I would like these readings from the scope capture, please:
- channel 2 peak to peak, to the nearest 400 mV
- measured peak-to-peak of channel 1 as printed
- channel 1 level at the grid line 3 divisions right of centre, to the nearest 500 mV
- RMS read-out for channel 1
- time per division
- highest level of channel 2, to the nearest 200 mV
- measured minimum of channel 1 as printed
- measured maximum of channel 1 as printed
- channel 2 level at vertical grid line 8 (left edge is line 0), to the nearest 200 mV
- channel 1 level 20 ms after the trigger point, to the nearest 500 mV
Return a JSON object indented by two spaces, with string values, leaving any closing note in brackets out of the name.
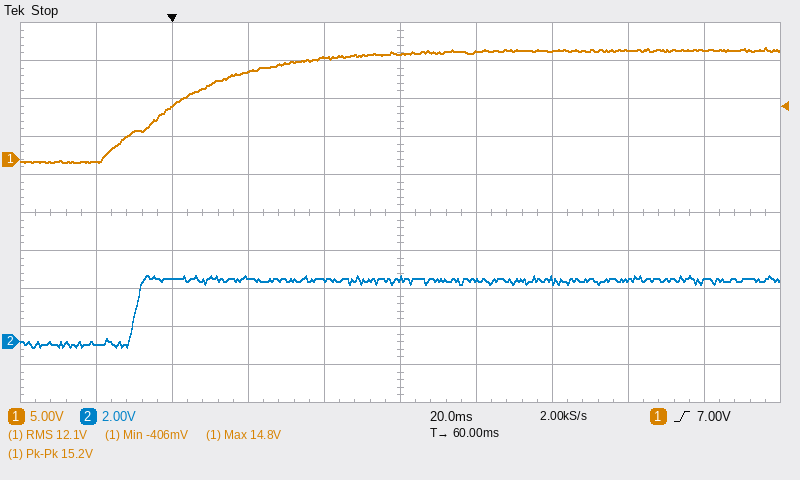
{
  "channel 2 peak to peak, to the nearest 400 mV": "3.6 V",
  "measured peak-to-peak of channel 1 as printed": "15.2 V",
  "channel 1 level at the grid line 3 divisions right of centre, to the nearest 500 mV": "14.5 V",
  "RMS read-out for channel 1": "12.1 V",
  "time per division": "20 ms",
  "highest level of channel 2, to the nearest 200 mV": "3.4 V",
  "measured minimum of channel 1 as printed": "-406 mV",
  "measured maximum of channel 1 as printed": "14.8 V",
  "channel 2 level at vertical grid line 8 (left edge is line 0), to the nearest 200 mV": "3.2 V",
  "channel 1 level 20 ms after the trigger point, to the nearest 500 mV": "11.5 V"
}
